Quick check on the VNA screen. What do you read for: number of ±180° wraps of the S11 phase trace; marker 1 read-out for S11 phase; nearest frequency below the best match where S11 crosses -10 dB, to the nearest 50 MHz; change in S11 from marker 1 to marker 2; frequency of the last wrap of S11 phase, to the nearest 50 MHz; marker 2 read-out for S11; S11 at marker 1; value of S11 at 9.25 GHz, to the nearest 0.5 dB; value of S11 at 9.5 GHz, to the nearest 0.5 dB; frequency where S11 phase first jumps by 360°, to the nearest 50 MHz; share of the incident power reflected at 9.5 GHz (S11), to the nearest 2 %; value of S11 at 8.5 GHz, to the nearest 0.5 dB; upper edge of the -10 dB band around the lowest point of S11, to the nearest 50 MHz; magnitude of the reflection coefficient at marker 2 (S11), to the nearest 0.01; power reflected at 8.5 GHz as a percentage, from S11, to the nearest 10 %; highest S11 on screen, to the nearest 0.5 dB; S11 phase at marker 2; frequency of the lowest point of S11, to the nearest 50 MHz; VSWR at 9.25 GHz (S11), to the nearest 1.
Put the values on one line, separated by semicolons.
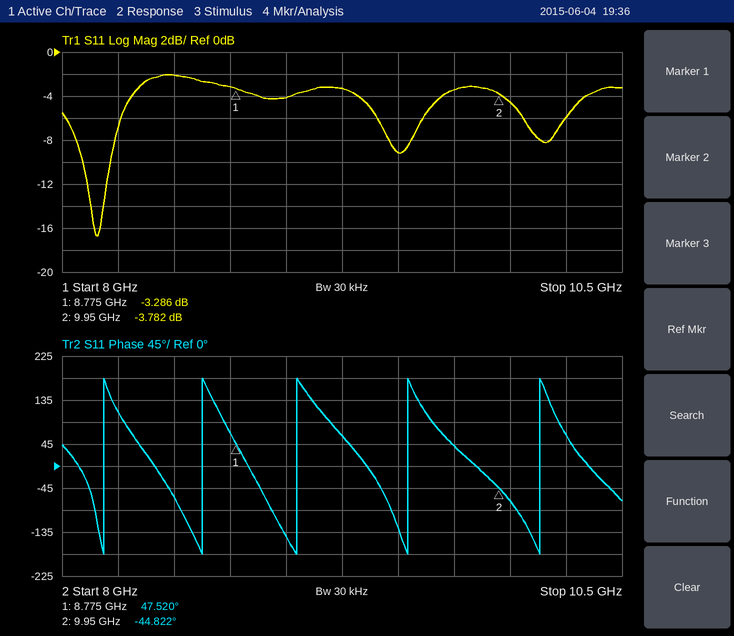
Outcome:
5; 47.520°; 8.10 GHz; -0.496 dB; 10.15 GHz; -3.782 dB; -3.286 dB; -3.5 dB; -9.0 dB; 8.20 GHz; 12 %; -2.0 dB; 8.20 GHz; 0.65; 60 %; -2.0 dB; -44.822°; 8.15 GHz; 5
